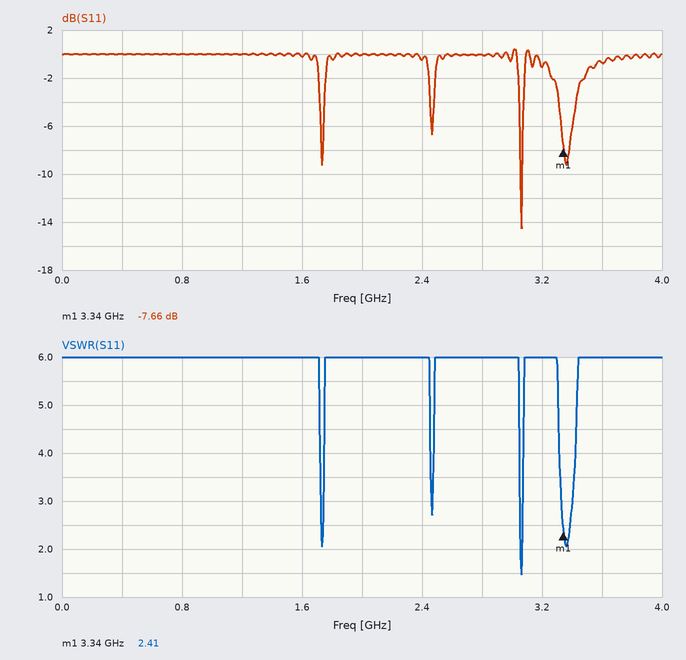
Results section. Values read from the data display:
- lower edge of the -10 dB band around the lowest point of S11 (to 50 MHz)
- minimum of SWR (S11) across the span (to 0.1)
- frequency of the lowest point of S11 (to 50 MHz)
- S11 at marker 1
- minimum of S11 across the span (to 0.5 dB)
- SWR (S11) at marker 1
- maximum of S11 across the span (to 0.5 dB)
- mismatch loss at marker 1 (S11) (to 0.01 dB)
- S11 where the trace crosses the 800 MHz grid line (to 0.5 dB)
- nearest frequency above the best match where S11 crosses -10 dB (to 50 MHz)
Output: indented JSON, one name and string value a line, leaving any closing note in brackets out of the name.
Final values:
{
  "lower edge of the -10 dB band around the lowest point of S11": "3.05 GHz",
  "minimum of SWR (S11) across the span": "1.5",
  "frequency of the lowest point of S11": "3.05 GHz",
  "S11 at marker 1": "-7.66 dB",
  "minimum of S11 across the span": "-14.5 dB",
  "SWR (S11) at marker 1": "2.41",
  "maximum of S11 across the span": "0.5 dB",
  "mismatch loss at marker 1 (S11)": "0.82 dB",
  "S11 where the trace crosses the 800 MHz grid line": "0.0 dB",
  "nearest frequency above the best match where S11 crosses -10 dB": "3.05 GHz"
}
